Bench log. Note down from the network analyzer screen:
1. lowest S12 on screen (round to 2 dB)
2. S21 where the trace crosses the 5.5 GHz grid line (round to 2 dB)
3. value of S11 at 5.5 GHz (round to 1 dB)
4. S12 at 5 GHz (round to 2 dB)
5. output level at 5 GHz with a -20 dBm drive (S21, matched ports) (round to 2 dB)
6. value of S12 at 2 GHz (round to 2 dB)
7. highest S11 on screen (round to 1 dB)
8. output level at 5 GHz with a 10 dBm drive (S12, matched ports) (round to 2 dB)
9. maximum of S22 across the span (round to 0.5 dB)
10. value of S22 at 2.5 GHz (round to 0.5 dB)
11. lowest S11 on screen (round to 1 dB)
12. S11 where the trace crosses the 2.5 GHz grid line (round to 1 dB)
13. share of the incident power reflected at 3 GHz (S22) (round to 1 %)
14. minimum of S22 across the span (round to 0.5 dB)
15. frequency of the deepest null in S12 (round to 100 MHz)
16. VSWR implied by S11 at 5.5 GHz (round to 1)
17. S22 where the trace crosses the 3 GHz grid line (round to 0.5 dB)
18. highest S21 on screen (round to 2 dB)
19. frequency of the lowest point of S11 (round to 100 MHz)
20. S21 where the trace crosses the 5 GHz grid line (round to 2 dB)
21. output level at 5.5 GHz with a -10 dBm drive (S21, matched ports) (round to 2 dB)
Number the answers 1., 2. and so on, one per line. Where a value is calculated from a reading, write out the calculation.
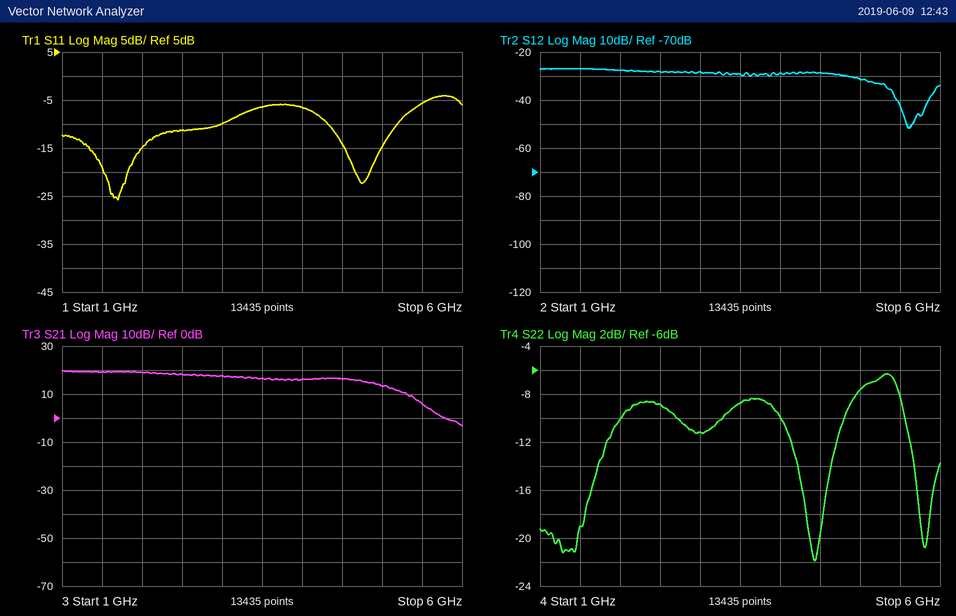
1. -52 dB
2. 6 dB
3. -6 dB
4. -32 dB
5. -20 dBm + (14 dB) = -6 dBm
6. -28 dB
7. -4 dB
8. 10 dBm + (-32 dB) = -22 dBm
9. -6.5 dB
10. -9.0 dB
11. -26 dB
12. -11 dB
13. 10^(-11/10) ≈ 8 %
14. -22.0 dB
15. 5.6 GHz
16. |Γ| = 10^(-6/20) = 0.5012; VSWR = (1 + 0.5012)/(1 − 0.5012) ≈ 3
17. -11.0 dB
18. 20 dB
19. 1.7 GHz
20. 14 dB
21. -10 dBm + (6 dB) = -4 dBm
